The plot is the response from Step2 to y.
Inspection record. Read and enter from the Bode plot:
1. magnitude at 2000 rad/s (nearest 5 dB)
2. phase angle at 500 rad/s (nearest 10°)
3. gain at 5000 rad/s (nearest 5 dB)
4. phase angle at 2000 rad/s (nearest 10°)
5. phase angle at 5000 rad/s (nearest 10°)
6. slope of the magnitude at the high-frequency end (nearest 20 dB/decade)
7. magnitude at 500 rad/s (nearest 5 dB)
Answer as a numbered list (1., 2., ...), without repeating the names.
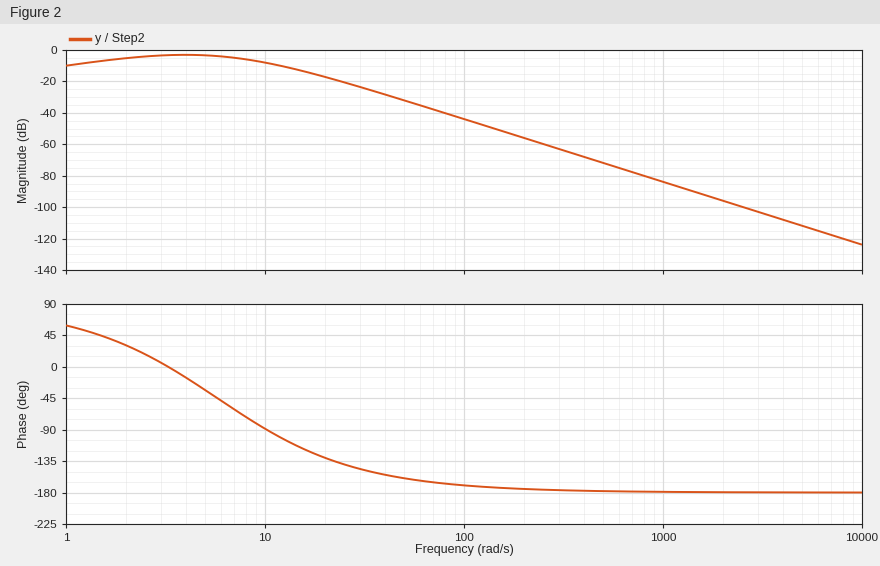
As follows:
1. -95 dB
2. -180°
3. -110 dB
4. -180°
5. -180°
6. -40 dB/decade
7. -70 dB
